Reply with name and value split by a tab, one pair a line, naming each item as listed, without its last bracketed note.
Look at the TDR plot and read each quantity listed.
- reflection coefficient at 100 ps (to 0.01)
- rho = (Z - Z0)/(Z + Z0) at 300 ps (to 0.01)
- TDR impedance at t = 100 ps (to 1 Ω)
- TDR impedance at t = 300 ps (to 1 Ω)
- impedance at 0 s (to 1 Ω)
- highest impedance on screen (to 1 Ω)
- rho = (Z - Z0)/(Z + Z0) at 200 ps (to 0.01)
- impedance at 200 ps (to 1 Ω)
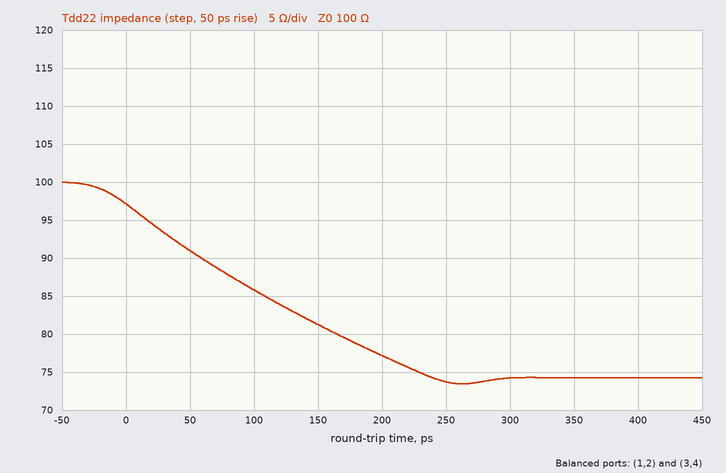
reflection coefficient at 100 ps	-0.08
rho = (Z - Z0)/(Z + Z0) at 300 ps	-0.15
TDR impedance at t = 100 ps	86 Ω
TDR impedance at t = 300 ps	74 Ω
impedance at 0 s	97 Ω
highest impedance on screen	100 Ω
rho = (Z - Z0)/(Z + Z0) at 200 ps	-0.13
impedance at 200 ps	77 Ω
